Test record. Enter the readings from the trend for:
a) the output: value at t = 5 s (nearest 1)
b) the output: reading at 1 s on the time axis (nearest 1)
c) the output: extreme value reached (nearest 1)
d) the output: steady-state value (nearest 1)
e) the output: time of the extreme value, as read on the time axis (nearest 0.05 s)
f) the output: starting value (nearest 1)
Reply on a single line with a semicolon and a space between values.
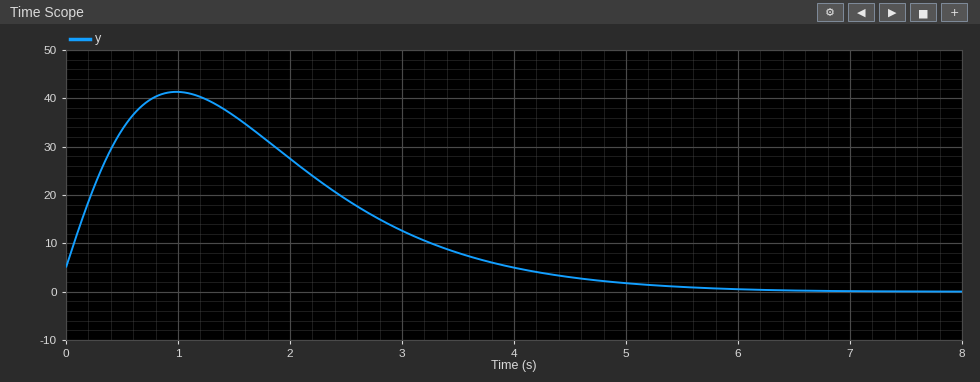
2; 41; 41; 0; 1.00 s; 5
